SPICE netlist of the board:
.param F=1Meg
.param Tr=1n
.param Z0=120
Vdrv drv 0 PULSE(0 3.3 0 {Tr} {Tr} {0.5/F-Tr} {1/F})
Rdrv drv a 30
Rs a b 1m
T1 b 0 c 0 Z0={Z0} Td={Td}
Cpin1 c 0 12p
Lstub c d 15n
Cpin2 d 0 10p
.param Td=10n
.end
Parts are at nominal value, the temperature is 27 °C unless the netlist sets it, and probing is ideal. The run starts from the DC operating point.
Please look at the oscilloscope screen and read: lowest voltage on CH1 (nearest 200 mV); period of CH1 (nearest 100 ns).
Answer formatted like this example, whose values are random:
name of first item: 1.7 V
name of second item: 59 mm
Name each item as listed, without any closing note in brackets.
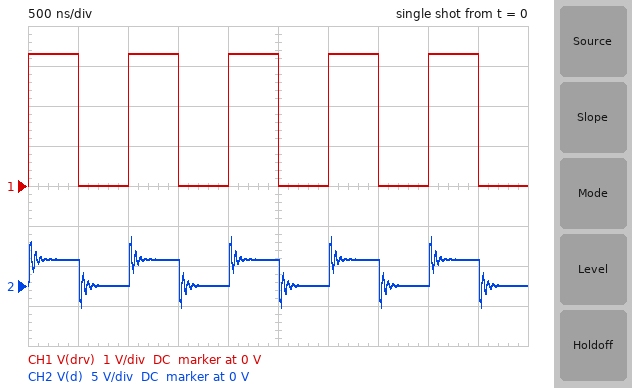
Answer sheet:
lowest voltage on CH1: 0 V
period of CH1: 1.0 µs
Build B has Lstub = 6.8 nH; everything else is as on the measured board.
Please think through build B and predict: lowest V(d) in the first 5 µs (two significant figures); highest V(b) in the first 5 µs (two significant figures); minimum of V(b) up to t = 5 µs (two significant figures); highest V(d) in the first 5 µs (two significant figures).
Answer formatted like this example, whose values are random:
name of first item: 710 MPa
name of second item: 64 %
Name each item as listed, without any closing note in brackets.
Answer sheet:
lowest V(d) in the first 5 µs: -2.7 V
highest V(b) in the first 5 µs: 4.0 V
minimum of V(b) up to t = 5 µs: -700 mV
highest V(d) in the first 5 µs: 6.0 V
